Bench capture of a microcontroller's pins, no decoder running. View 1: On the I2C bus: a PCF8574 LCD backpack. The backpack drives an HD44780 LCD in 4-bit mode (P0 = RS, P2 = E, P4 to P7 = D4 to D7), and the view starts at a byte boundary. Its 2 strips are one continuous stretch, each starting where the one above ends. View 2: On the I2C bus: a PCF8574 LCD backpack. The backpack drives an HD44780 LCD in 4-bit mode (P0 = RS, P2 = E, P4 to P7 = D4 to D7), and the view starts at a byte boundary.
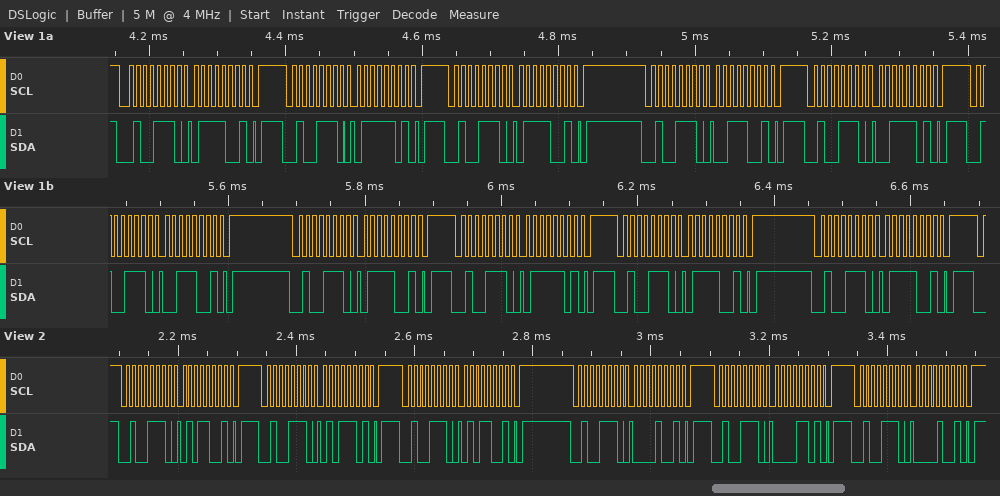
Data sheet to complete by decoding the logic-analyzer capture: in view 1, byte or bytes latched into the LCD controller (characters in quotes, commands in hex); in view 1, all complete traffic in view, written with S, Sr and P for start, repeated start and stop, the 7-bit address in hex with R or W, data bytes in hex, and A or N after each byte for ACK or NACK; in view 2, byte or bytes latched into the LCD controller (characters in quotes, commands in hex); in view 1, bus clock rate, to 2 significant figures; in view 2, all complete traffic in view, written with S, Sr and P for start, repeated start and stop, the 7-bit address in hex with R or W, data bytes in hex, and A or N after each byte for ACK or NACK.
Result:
's'
S 27W A 79 A P S 27W A 7D A P S 27W A 79 A P S 27W A 39 A P S 27W A 3D A P S 27W A 39 A P S 27W A 79 A P S 27W A 7D A P S 27W A 79 A P S 27W A 79 A P
'P'
100 kHz
S 27W A 59 A P S 27W A 5D A P S 27W A 59 A P S 27W A 09 A P S 27W A 0D A P S 27W A 09 A P
